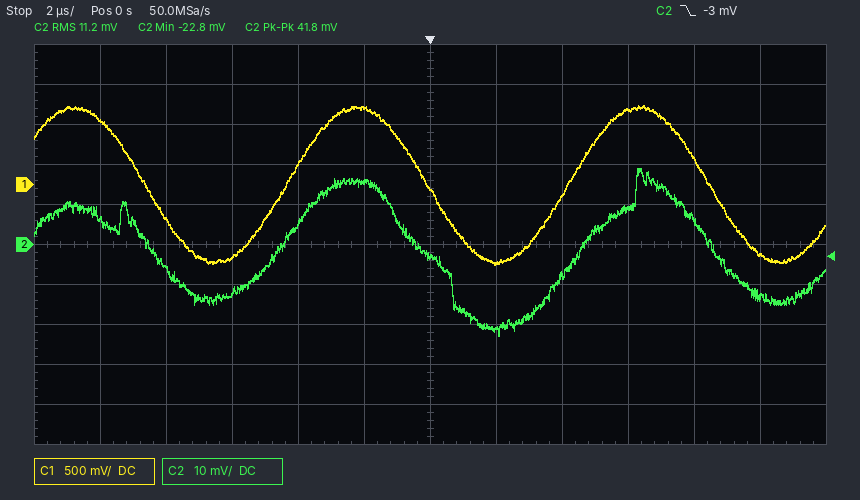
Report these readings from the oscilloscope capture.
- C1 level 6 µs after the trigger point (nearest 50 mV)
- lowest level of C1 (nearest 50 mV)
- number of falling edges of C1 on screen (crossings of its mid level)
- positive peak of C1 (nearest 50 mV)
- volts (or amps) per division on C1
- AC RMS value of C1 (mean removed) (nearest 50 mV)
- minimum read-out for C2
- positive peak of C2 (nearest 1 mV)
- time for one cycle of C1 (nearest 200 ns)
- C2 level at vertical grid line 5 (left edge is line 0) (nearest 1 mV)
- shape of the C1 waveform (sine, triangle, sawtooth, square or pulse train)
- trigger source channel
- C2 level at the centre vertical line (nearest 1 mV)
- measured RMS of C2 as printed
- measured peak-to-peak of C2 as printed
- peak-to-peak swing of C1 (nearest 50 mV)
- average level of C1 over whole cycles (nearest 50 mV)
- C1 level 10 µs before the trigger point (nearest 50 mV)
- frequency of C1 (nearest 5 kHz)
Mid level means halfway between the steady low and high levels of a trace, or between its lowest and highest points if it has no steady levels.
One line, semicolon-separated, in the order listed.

950 mV; -1.00 V; 3; 1.00 V; 500 mV; 700 mV; -22.8 mV; 19 mV; 8.6 µs; 16 mV; sine; C2; -3 mV; 11.2 mV; 41.8 mV; 2.00 V; 0 mV; 800 mV; 115 kHz
